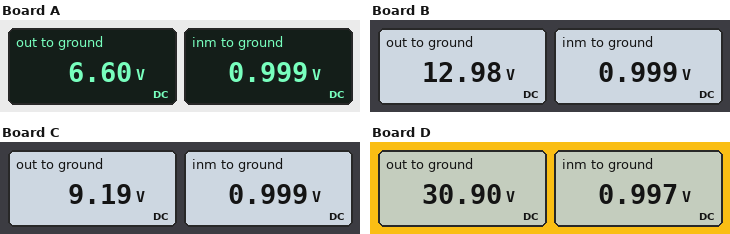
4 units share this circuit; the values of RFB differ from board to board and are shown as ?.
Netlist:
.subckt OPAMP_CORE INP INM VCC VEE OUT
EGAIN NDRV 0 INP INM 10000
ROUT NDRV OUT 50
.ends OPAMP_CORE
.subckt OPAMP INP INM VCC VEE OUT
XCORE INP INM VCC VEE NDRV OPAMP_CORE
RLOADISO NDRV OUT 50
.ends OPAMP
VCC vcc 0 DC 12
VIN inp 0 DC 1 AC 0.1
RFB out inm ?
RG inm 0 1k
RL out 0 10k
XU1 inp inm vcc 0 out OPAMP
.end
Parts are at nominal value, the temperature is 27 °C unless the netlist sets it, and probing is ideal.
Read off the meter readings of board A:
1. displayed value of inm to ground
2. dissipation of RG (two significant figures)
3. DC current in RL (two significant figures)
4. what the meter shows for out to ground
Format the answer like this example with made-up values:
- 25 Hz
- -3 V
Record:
- 0.999 V
- 1.0 mW
- 660 µA
- 6.60 V
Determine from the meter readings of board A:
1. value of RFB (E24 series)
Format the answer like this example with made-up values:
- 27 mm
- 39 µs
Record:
- 5.6 kΩ
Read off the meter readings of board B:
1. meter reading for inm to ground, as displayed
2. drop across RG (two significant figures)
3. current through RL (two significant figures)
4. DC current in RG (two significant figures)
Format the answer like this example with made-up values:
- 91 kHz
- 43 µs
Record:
- 0.999 V
- 1.0 V
- 1.3 mA
- 1.0 mA
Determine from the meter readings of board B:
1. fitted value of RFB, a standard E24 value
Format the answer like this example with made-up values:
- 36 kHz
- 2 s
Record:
- 12 kΩ
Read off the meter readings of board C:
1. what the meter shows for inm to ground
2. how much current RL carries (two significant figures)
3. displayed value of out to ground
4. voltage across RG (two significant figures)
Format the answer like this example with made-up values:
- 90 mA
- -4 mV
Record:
- 0.999 V
- 920 µA
- 9.19 V
- 1.0 V
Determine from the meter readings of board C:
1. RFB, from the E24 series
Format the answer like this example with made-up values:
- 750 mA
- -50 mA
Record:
- 8.2 kΩ
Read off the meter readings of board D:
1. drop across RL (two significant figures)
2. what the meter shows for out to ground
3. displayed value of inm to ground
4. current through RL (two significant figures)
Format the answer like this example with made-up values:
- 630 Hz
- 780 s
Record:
- 31 V
- 30.90 V
- 0.997 V
- 3.1 mA
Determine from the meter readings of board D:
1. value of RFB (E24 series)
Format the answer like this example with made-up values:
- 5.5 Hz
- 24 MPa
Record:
- 30 kΩ
